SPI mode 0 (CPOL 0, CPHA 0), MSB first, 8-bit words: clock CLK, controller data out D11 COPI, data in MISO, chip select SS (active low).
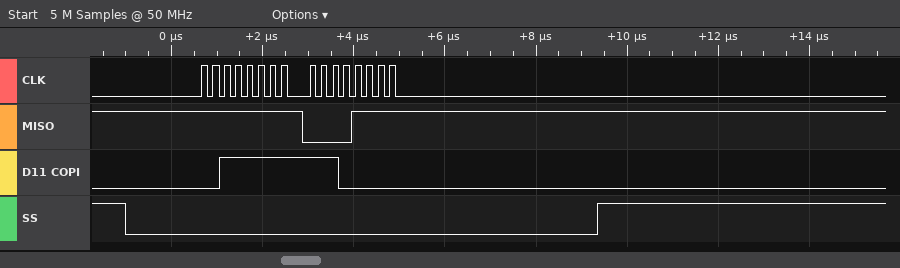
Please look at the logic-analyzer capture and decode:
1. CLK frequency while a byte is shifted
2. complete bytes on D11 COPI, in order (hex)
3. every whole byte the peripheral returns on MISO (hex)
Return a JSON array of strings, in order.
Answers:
["4 MHz", "0x3F 0xE0", "0xFF 0x0F"]
